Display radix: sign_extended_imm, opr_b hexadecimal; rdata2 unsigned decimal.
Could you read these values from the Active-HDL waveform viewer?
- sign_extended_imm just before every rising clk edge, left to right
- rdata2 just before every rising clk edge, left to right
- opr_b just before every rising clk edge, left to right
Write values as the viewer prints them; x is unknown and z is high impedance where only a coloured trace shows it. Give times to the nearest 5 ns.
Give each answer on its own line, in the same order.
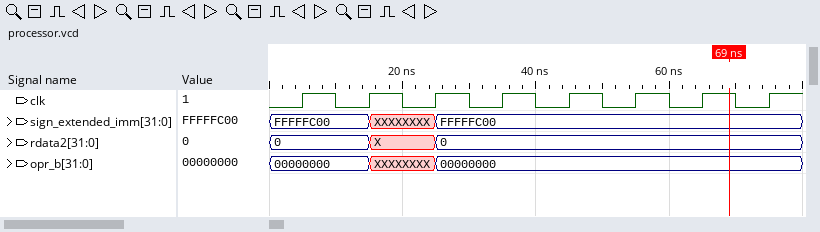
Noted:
FFFFFC00, FFFFFC00, XXXXXXXX, FFFFFC00, FFFFFC00, FFFFFC00, FFFFFC00, FFFFFC00
0, 0, X, 0, 0, 0, 0, 0
00000000, 00000000, XXXXXXXX, 00000000, 00000000, 00000000, 00000000, 00000000
